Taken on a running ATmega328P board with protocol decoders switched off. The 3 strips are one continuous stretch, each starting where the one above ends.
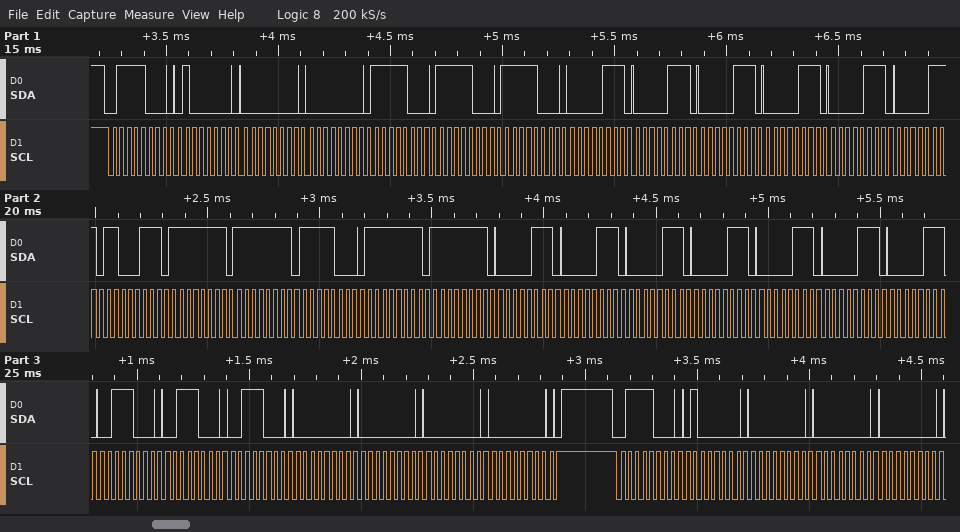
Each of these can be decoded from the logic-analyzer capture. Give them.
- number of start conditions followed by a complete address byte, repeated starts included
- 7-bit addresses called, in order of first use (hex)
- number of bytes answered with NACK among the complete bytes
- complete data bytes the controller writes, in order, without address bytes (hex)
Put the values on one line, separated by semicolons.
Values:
2; 0x3C; 0; 40 00 00 F8 F8 F8 07 07 07 07 07 07 C7 FF FF F8 FF FF 07 07 07 07 07 07 07 38 38 38 00 00 00 00 40 00 00 00
